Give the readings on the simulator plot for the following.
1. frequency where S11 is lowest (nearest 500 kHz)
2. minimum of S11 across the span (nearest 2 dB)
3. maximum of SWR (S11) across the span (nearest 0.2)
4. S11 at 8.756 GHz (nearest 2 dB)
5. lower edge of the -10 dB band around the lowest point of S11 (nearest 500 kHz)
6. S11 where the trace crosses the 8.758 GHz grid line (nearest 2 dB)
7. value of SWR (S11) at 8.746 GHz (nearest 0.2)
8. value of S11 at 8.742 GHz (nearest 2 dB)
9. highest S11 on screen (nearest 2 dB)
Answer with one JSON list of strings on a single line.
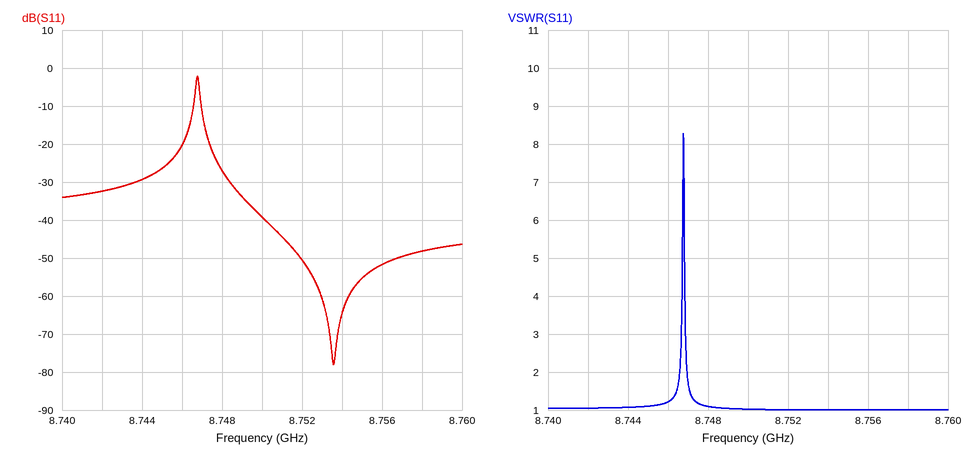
["8.7535 GHz", "-78 dB", "8.2", "-52 dB", "8.7470 GHz", "-48 dB", "1.2", "-32 dB", "-2 dB"]
